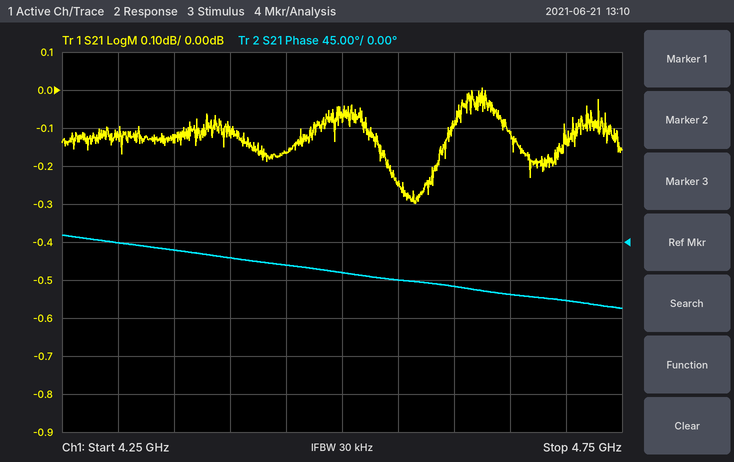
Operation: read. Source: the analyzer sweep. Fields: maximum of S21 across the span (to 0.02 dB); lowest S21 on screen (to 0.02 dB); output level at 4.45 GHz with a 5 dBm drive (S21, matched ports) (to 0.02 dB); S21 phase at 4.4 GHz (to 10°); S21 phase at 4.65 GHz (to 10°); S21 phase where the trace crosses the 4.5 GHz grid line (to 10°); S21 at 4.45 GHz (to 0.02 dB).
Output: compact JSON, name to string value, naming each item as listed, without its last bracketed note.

{"maximum of S21 across the span": "0.00 dB", "lowest S21 on screen": "-0.30 dB", "output level at 4.45 GHz with a 5 dBm drive (S21, matched ports)": "4.84 dBm", "S21 phase at 4.4 GHz": "-20°", "S21 phase at 4.65 GHz": "-60°", "S21 phase where the trace crosses the 4.5 GHz grid line": "-40°", "S21 at 4.45 GHz": "-0.16 dB"}
